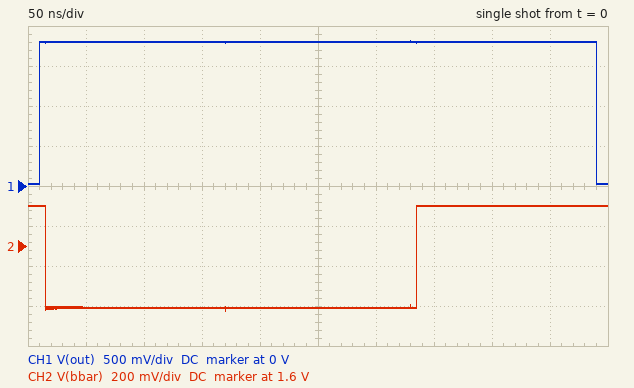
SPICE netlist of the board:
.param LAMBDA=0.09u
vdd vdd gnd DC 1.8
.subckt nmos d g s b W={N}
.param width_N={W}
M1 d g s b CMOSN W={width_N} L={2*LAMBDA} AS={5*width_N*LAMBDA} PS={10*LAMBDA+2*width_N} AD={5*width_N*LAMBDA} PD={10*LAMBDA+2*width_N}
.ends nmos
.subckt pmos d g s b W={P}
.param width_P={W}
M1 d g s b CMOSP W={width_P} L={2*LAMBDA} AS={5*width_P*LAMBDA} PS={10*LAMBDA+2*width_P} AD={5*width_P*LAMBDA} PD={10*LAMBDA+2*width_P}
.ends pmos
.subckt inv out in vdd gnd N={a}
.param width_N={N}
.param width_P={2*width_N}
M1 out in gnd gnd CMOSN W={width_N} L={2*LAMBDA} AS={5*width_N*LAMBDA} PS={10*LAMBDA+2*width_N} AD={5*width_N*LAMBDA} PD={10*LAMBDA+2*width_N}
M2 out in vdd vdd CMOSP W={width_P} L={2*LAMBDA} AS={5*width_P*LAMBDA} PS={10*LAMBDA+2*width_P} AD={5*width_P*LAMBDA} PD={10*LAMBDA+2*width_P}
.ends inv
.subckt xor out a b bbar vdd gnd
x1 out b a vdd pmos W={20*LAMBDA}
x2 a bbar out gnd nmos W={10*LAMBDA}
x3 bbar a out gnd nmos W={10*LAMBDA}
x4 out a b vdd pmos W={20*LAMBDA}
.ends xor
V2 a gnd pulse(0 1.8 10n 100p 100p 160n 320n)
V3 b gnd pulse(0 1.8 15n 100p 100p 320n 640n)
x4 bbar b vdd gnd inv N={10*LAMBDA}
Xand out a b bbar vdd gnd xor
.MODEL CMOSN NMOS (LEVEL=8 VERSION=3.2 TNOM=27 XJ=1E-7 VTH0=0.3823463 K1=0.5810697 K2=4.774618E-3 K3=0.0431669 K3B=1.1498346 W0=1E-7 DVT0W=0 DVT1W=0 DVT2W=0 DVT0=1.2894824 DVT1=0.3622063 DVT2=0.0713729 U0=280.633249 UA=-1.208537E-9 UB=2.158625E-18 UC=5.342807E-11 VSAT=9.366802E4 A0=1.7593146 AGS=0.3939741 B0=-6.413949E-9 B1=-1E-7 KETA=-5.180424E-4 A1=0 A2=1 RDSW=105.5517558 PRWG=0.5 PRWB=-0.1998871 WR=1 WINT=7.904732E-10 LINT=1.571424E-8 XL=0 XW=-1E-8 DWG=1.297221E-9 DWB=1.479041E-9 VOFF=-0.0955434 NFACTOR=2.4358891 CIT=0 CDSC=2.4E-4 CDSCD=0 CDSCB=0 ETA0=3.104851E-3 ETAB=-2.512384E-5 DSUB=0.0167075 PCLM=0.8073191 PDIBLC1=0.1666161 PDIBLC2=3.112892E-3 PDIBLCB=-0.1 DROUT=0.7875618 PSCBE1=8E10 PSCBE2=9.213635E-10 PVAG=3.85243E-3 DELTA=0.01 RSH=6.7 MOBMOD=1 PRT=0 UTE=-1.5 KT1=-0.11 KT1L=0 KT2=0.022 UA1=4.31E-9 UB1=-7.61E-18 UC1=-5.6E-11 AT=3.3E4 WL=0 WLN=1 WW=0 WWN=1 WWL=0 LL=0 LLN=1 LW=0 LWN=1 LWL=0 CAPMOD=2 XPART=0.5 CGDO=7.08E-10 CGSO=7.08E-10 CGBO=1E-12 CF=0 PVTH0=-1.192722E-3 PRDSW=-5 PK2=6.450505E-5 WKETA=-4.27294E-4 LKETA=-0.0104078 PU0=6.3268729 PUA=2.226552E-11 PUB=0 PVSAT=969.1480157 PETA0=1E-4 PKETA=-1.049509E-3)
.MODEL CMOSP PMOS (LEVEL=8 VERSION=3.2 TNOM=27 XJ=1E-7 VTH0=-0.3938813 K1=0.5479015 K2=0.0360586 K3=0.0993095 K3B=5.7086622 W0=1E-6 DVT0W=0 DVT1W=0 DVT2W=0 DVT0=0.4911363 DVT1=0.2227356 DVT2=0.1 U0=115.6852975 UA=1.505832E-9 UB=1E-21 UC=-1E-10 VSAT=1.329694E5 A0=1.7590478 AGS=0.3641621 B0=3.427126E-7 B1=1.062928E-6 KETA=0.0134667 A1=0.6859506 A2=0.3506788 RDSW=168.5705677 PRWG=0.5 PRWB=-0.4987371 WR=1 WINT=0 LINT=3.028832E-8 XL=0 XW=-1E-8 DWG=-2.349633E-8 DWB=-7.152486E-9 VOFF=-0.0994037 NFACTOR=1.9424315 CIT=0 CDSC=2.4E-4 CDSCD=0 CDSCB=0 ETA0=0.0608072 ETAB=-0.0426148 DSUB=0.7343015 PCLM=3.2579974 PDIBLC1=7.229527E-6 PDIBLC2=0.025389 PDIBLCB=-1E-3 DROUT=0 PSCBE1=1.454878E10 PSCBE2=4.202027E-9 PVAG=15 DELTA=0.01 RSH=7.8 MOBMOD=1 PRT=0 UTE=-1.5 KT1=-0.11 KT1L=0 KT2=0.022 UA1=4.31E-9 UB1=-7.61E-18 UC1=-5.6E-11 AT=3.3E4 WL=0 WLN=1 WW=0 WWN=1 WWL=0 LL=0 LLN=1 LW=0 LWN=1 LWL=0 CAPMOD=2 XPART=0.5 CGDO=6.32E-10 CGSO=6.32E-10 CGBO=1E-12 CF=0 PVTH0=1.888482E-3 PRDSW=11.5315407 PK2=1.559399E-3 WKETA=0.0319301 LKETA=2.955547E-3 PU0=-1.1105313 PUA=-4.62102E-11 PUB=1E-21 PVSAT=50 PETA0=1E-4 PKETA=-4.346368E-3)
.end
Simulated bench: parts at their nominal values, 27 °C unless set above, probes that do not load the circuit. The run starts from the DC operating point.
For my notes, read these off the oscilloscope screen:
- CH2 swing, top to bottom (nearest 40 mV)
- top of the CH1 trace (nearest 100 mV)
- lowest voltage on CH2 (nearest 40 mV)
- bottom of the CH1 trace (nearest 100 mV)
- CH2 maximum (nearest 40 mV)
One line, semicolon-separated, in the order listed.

520 mV; 1.8 V; 1.28 V; 0 V; 1.80 V
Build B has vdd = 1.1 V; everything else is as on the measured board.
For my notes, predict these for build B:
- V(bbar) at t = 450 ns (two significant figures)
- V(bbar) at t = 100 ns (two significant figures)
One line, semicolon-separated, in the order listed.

1.1 V; 550 mV
